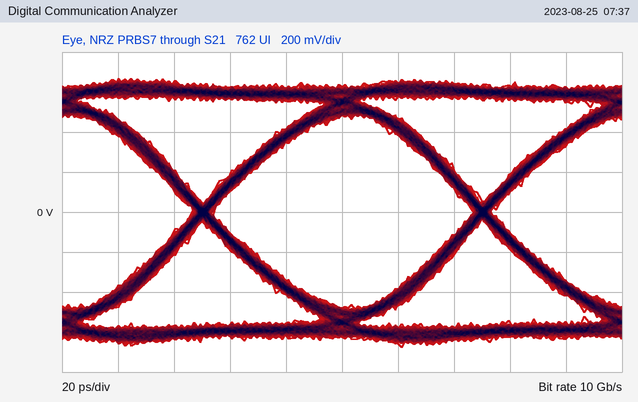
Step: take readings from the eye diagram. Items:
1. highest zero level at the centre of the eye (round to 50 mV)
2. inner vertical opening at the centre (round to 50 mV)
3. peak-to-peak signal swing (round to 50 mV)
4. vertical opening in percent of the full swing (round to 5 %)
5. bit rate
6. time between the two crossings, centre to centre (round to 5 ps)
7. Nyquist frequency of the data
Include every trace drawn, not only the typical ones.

-500 mV
950 mV
1.35 V
70 %
10 Gb/s
100 ps
5 GHz
